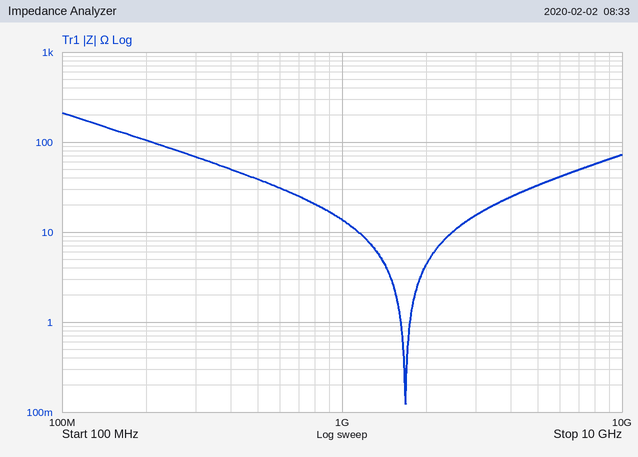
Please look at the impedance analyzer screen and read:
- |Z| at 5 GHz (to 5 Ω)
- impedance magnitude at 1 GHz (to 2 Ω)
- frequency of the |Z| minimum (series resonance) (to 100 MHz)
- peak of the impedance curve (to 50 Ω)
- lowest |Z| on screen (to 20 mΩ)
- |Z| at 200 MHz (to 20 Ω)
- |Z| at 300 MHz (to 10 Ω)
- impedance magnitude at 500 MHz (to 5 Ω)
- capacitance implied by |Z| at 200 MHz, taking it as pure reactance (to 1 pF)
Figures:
35 Ω
14 Ω
1.7 GHz
200 Ω
120 mΩ
100 Ω
70 Ω
40 Ω
8 pF
